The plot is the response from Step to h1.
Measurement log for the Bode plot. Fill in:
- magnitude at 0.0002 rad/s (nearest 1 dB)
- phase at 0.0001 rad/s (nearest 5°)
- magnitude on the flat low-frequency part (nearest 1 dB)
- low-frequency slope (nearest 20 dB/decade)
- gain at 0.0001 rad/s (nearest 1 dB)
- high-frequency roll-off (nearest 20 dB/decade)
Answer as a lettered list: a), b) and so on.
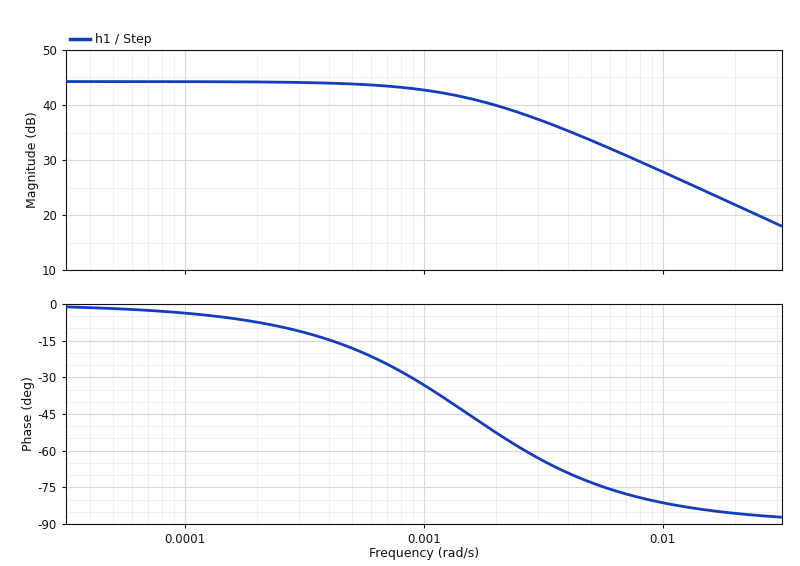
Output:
a) 44 dB
b) -5°
c) 44 dB
d) 0 dB/decade
e) 44 dB
f) -20 dB/decade
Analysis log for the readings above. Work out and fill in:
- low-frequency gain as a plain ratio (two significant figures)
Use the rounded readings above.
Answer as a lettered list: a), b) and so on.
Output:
a) 160
